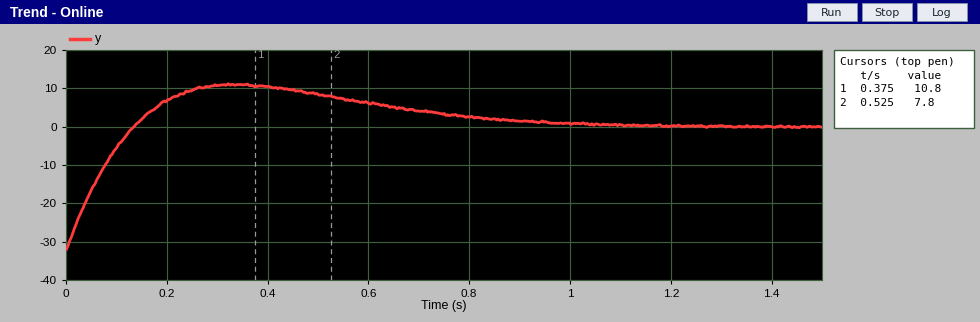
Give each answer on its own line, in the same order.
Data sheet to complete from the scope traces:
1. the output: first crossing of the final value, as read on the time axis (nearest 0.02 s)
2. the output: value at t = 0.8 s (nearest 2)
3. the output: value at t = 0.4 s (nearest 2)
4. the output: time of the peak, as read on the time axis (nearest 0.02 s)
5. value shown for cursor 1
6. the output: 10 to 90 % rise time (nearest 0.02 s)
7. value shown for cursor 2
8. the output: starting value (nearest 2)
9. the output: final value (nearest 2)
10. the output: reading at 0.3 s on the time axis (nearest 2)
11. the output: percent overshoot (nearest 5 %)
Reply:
0.14 s
2
10
0.34 s
10.8
0.10 s
7.8
-32
0
10
35 %
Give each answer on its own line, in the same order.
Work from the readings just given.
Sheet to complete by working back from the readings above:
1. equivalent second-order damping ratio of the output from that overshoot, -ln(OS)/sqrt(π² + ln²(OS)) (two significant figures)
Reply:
0.32
